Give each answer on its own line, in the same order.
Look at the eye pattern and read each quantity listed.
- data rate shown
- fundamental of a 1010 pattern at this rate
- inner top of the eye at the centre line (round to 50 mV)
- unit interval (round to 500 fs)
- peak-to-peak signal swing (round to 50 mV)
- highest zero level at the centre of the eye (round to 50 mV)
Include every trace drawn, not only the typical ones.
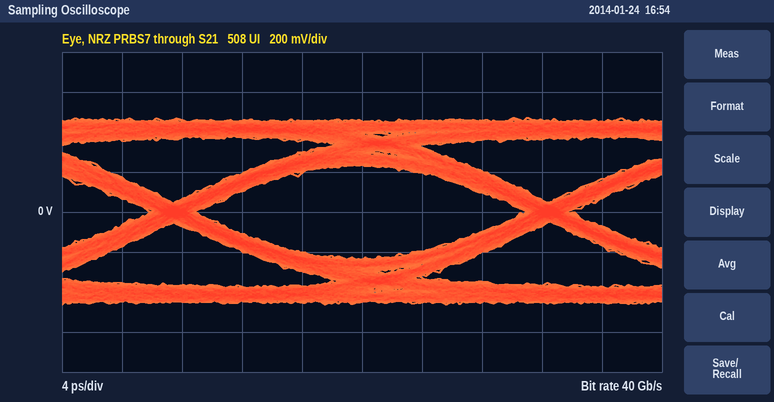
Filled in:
40 Gb/s
20 GHz
250 mV
25.0 ps
950 mV
-250 mV
